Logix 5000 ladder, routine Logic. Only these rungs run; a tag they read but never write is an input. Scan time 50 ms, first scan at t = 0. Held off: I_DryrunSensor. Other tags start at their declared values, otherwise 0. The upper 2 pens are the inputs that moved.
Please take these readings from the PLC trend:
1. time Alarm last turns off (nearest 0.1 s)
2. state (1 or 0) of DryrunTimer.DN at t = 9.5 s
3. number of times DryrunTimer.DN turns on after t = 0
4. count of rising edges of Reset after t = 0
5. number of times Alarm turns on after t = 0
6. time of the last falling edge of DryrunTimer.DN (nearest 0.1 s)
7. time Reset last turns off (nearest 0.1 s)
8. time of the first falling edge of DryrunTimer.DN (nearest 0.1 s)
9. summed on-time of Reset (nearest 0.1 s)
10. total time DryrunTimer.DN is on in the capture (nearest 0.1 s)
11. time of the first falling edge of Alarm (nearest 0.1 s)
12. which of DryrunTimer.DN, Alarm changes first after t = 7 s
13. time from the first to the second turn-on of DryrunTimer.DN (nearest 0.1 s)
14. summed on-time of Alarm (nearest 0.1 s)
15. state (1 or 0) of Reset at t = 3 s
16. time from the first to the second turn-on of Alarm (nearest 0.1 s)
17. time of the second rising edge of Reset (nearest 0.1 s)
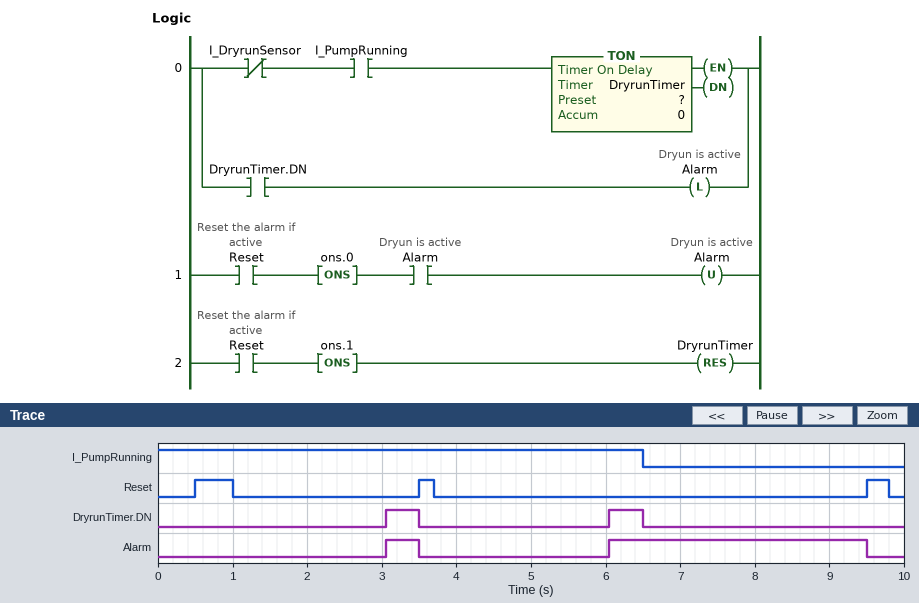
9.5 s
0
2
3
2
6.5 s
9.8 s
3.5 s
1.0 s
0.9 s
3.5 s
Alarm
3.0 s
3.9 s
0
3.0 s
3.5 s
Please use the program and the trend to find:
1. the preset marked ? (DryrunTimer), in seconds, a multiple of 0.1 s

2.5 s
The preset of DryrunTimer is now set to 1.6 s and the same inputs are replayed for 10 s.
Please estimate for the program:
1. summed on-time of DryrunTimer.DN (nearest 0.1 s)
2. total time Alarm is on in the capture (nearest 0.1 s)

2.7 s
5.7 s
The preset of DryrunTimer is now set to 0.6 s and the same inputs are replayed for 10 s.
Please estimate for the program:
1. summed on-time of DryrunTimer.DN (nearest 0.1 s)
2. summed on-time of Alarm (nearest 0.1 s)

4.7 s
7.7 s
